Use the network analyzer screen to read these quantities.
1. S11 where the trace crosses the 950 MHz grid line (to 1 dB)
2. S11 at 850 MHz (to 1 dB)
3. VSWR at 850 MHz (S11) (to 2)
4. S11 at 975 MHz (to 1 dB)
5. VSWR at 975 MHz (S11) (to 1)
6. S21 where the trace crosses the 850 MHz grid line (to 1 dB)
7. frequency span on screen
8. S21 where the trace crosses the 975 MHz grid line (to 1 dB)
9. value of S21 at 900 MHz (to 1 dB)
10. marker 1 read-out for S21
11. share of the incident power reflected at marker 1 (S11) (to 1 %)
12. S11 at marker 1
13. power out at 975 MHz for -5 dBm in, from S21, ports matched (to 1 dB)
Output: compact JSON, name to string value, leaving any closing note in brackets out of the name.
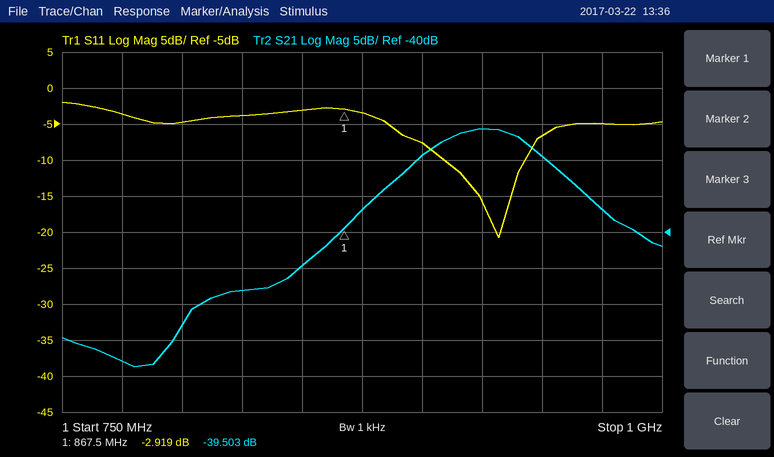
{"S11 where the trace crosses the 950 MHz grid line": "-7 dB", "S11 at 850 MHz": "-3 dB", "VSWR at 850 MHz (S11)": "6", "S11 at 975 MHz": "-5 dB", "VSWR at 975 MHz (S11)": "4", "S21 where the trace crosses the 850 MHz grid line": "-45 dB", "frequency span on screen": "250 MHz", "S21 where the trace crosses the 975 MHz grid line": "-37 dB", "value of S21 at 900 MHz": "-29 dB", "marker 1 read-out for S21": "-39.503 dB", "share of the incident power reflected at marker 1 (S11)": "51 %", "S11 at marker 1": "-2.919 dB", "power out at 975 MHz for -5 dBm in, from S21, ports matched": "-42 dBm"}
